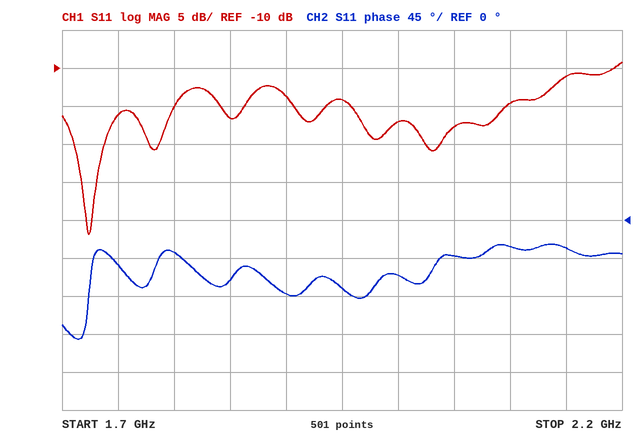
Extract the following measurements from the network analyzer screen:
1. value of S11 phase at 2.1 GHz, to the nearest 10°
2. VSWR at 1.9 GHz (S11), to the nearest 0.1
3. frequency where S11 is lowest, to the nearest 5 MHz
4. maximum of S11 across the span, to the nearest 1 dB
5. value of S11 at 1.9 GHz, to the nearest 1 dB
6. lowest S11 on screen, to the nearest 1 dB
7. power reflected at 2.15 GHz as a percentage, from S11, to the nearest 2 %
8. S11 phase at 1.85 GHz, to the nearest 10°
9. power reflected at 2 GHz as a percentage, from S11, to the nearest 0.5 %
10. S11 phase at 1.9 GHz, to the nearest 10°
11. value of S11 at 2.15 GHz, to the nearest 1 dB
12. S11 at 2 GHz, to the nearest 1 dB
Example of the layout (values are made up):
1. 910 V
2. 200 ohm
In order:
1. -30°
2. 1.5
3. 1.725 GHz
4. -9 dB
5. -14 dB
6. -32 dB
7. 8 %
8. -70°
9. 2.0 %
10. -90°
11. -11 dB
12. -17 dB
